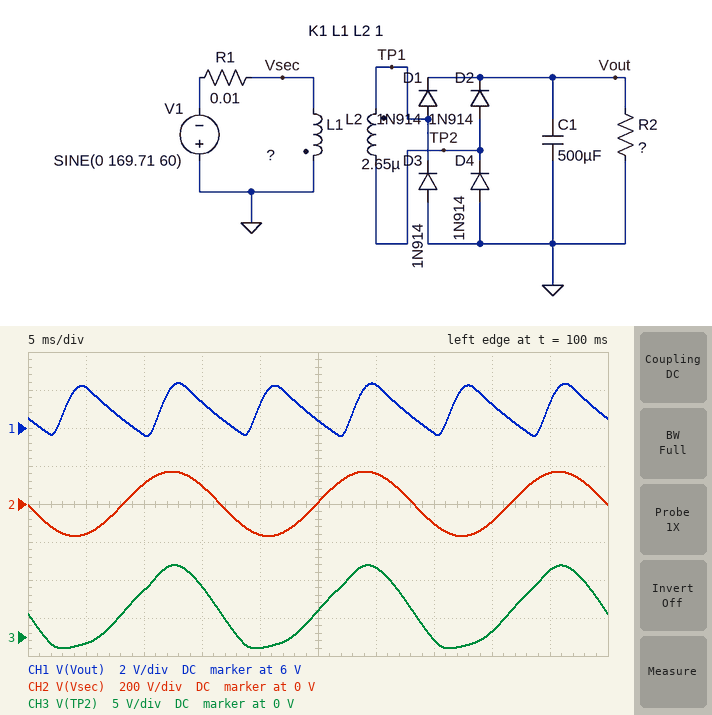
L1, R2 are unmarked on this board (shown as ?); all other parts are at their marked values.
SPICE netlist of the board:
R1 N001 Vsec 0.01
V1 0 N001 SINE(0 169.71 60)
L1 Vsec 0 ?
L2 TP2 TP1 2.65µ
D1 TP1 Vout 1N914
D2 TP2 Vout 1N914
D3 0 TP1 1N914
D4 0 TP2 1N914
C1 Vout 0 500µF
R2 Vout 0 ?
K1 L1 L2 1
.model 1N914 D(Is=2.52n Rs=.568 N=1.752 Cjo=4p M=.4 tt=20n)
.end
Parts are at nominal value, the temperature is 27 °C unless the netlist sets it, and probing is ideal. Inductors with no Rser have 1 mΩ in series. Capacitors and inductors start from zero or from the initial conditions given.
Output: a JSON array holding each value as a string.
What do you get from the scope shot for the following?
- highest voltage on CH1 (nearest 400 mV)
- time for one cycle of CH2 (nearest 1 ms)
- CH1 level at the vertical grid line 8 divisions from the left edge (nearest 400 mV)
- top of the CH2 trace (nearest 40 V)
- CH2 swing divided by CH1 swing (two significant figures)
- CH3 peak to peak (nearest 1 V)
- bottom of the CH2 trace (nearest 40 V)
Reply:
["8.4 V", "17 ms", "7.2 V", "160 V", "120", "11 V", "-160 V"]
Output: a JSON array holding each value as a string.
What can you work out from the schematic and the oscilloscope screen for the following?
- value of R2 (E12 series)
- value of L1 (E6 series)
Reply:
["27 Ω", "680 µH"]
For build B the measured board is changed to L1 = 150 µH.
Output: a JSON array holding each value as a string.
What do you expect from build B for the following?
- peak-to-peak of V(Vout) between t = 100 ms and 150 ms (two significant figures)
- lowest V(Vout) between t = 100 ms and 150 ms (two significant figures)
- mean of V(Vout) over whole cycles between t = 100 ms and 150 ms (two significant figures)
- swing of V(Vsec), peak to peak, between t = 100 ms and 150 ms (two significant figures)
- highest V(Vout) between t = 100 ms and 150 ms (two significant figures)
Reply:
["6.2 V", "13 V", "16 V", "330 V", "19 V"]
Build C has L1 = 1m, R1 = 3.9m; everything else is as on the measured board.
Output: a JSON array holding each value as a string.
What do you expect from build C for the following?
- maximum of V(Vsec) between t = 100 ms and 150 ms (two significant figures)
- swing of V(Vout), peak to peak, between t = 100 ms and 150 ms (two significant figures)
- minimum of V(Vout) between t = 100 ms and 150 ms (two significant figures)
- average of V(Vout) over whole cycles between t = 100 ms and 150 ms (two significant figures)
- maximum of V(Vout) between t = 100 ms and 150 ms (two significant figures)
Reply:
["170 V", "2.2 V", "4.4 V", "5.5 V", "6.6 V"]
